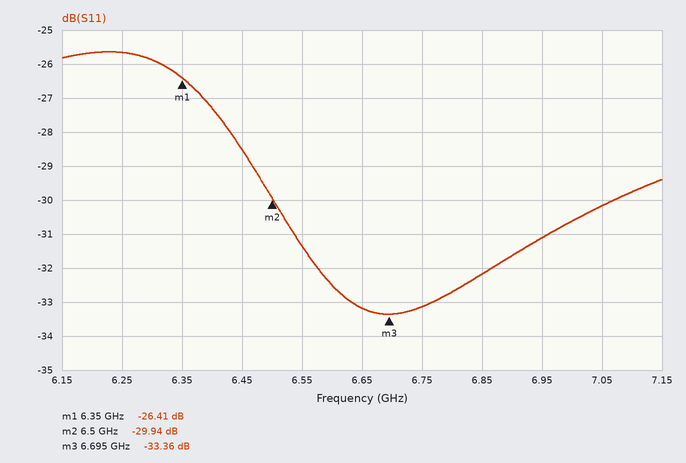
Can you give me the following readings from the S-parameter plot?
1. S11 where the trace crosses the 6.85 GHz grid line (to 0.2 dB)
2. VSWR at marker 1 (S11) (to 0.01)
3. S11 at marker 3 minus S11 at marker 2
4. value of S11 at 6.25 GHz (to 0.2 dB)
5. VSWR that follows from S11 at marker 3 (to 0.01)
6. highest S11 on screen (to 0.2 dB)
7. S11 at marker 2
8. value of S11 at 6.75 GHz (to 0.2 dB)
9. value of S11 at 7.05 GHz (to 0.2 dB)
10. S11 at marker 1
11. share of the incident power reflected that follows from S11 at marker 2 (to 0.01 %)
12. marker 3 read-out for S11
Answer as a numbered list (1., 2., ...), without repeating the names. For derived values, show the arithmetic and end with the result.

1. -32.2 dB
2. (1 + 0.0478)/(1 − 0.0478) ≈ 1.10
3. -33.36 − (-29.94) = -3.42 dB
4. -25.6 dB
5. (1 + 0.0215)/(1 − 0.0215) ≈ 1.04
6. -25.6 dB
7. -29.94 dB
8. -33.2 dB
9. -30.2 dB
10. -26.41 dB
11. 10^(-29.94/10) ≈ 0.10 %
12. -33.36 dB
